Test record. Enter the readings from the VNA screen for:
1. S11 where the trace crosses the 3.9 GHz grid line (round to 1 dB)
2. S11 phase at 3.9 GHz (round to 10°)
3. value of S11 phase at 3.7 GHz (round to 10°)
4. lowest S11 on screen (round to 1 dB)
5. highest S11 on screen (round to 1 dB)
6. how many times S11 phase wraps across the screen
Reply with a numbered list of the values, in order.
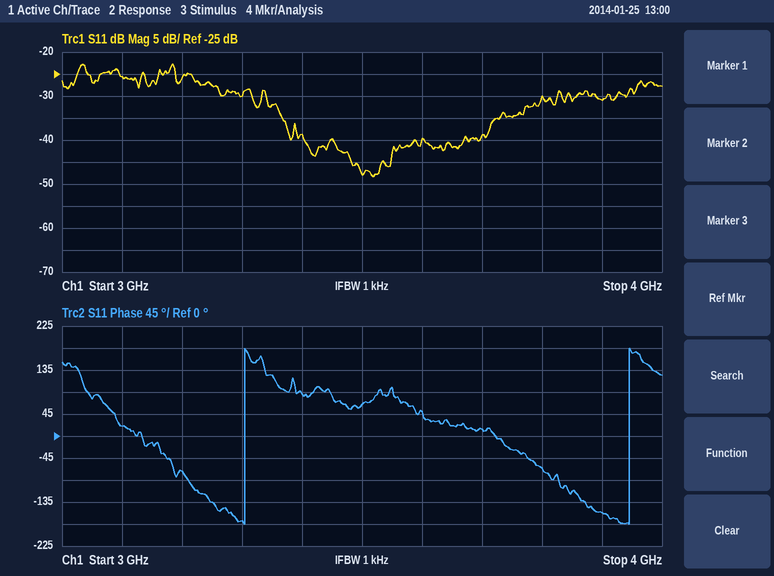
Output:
1. -31 dB
2. -160°
3. 10°
4. -48 dB
5. -23 dB
6. 2
